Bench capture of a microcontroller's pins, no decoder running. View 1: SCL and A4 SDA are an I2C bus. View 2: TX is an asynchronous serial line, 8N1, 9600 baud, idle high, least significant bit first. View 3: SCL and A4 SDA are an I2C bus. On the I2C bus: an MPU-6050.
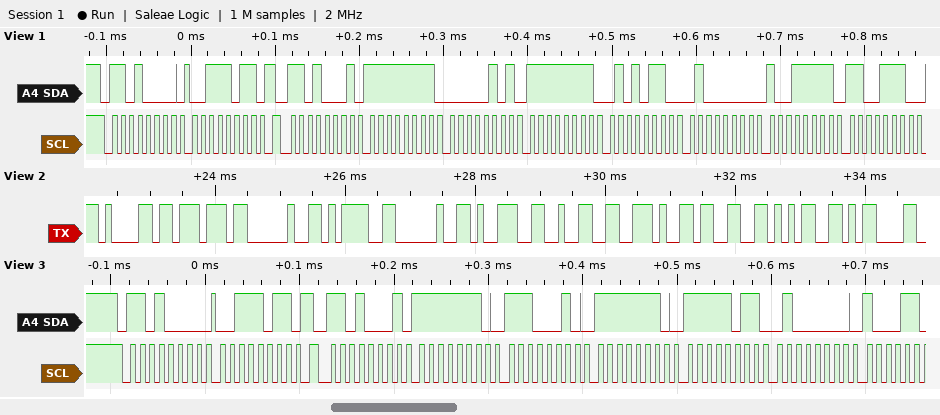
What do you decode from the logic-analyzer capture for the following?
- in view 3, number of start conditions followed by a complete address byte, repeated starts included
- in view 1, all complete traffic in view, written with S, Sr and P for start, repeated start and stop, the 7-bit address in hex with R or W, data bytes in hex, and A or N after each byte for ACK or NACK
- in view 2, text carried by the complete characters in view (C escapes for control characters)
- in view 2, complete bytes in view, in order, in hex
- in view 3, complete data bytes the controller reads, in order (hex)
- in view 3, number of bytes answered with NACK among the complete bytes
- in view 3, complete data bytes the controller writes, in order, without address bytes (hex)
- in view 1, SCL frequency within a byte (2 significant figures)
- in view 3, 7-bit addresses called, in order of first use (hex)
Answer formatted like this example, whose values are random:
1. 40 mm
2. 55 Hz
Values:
1. 2
2. S 68W A 3B A Sr 68R A FF A 05 A FF A 56 A 40 A 9F A CE A
3. "aw = 92.35\r"
4. 61 77 20 3D 20 39 32 2E 33 35 0D
5. FE E2 FE FB 40
6. 0
7. 3B
8. 100 kHz
9. 0x68
